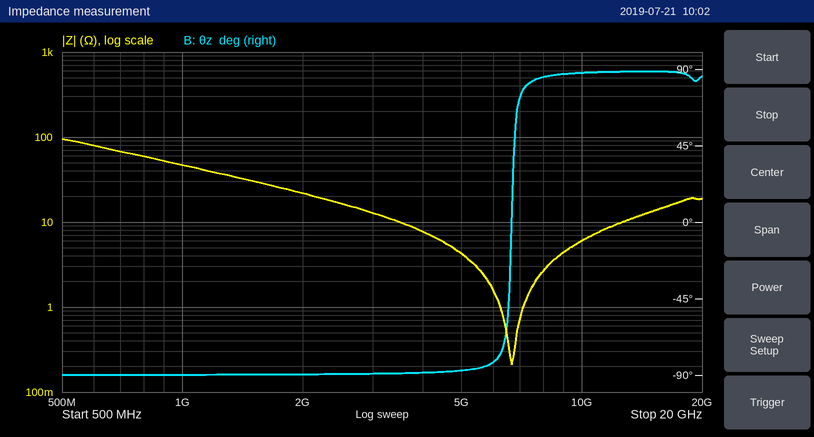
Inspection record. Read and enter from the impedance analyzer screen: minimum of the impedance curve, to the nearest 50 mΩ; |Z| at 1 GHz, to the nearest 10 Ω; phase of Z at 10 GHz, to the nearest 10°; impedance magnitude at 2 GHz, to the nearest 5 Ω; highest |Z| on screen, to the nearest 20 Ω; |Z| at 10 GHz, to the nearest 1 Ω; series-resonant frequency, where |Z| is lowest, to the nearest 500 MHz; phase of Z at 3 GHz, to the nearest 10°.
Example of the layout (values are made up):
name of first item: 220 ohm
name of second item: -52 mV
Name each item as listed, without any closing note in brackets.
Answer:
minimum of the impedance curve, to the nearest 50 mΩ: 200 mΩ
|Z| at 1 GHz, to the nearest 10 Ω: 50 Ω
phase of Z at 10 GHz, to the nearest 10°: 90°
impedance magnitude at 2 GHz, to the nearest 5 Ω: 20 Ω
highest |Z| on screen, to the nearest 20 Ω: 100 Ω
|Z| at 10 GHz, to the nearest 1 Ω: 6 Ω
series-resonant frequency, where |Z| is lowest, to the nearest 500 MHz: 6.5 GHz
phase of Z at 3 GHz, to the nearest 10°: -90°
